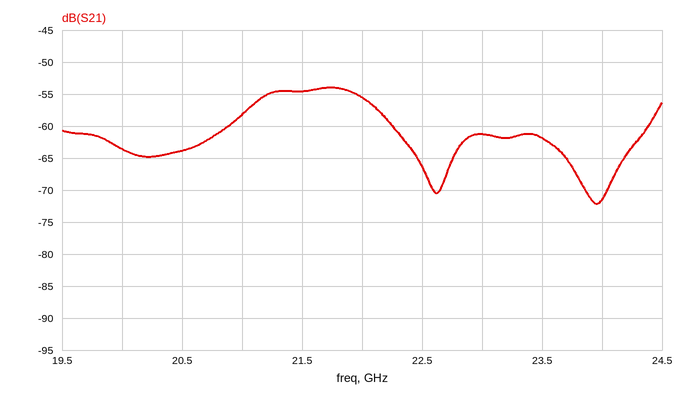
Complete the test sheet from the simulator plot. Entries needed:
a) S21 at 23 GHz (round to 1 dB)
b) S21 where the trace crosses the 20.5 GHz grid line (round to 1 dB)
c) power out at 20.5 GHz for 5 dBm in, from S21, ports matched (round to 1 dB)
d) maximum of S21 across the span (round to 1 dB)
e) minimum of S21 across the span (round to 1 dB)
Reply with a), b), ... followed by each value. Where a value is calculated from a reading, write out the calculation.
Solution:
a) -61 dB
b) -64 dB
c) 5 dBm + (-64 dB) = -59 dBm
d) -54 dB
e) -72 dB
